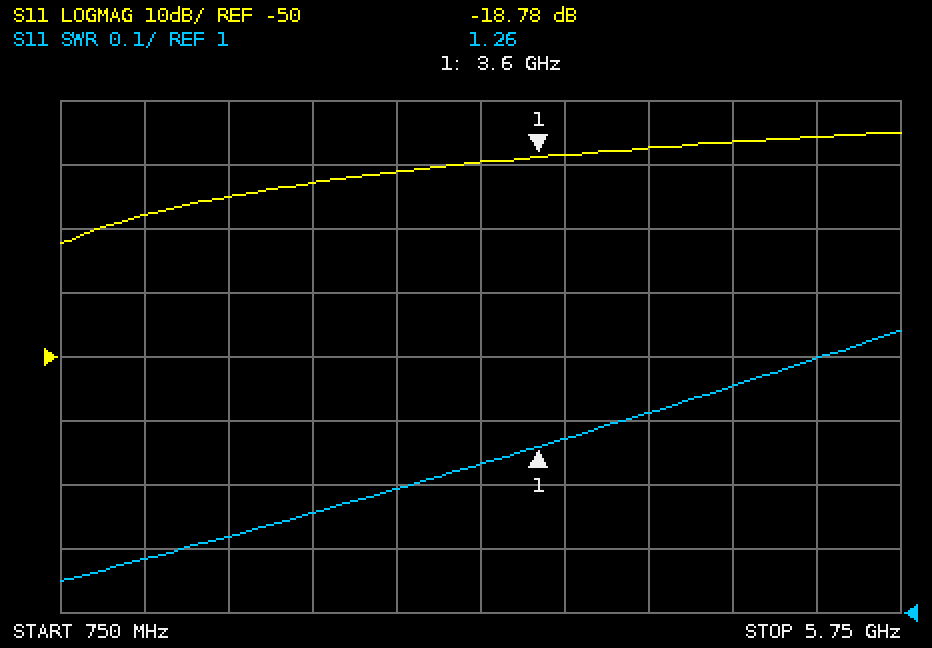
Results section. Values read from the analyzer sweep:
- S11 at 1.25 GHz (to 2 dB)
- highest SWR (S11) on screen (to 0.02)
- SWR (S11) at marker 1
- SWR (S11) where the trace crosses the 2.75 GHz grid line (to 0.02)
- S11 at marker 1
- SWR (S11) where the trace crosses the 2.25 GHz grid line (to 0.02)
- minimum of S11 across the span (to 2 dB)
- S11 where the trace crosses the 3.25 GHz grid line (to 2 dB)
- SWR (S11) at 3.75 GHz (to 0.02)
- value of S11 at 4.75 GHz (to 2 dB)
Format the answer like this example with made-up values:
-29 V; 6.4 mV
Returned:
-28 dB; 1.44; 1.26; 1.20; -18.78 dB; 1.16; -32 dB; -20 dB; 1.28; -16 dB
